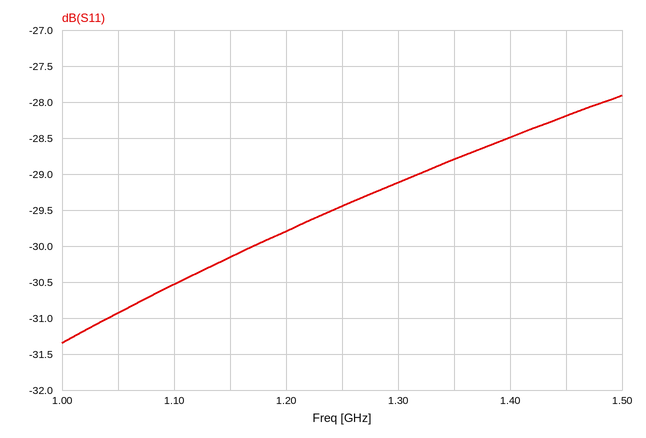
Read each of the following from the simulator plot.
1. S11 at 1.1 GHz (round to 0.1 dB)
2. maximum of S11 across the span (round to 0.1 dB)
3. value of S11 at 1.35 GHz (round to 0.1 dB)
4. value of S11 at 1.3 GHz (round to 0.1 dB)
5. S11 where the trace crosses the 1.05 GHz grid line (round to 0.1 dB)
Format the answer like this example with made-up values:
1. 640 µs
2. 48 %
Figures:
1. -30.5 dB
2. -27.9 dB
3. -28.8 dB
4. -29.1 dB
5. -30.9 dB
